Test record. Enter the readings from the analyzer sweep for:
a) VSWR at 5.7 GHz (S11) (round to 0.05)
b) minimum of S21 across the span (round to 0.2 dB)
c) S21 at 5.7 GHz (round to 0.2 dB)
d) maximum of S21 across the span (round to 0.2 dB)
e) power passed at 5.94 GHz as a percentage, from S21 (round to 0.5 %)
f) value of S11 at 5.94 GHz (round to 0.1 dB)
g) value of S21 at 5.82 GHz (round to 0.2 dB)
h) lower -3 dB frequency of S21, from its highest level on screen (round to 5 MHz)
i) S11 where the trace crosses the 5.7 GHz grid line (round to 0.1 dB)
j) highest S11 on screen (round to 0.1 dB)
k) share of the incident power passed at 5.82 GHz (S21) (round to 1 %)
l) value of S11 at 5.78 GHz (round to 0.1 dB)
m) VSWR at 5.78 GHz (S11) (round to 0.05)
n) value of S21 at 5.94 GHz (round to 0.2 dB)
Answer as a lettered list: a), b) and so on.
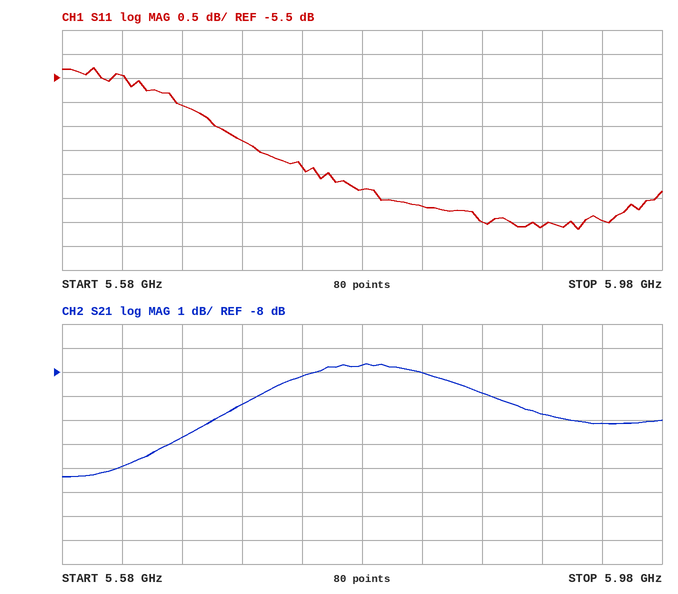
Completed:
a) 2.70
b) -12.4 dB
c) -9.4 dB
d) -7.6 dB
e) 9.5 %
f) -8.5 dB
g) -8.0 dB
h) 5.660 GHz
i) -6.8 dB
j) -5.3 dB
k) 16 %
l) -7.8 dB
m) 2.35
n) -10.2 dB
